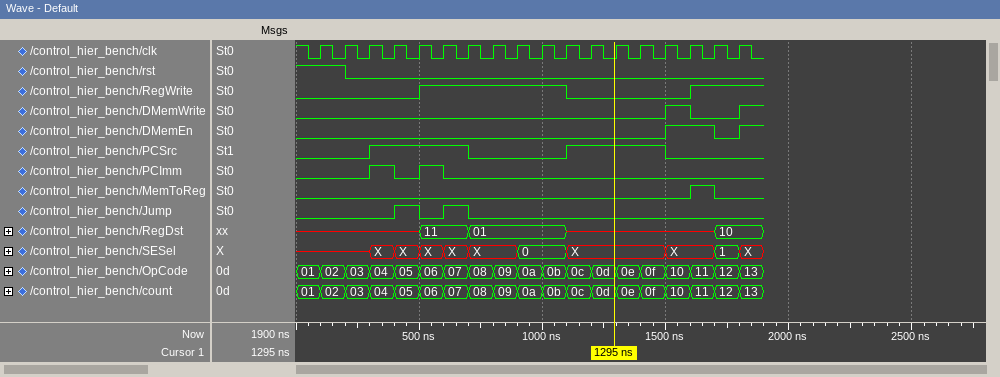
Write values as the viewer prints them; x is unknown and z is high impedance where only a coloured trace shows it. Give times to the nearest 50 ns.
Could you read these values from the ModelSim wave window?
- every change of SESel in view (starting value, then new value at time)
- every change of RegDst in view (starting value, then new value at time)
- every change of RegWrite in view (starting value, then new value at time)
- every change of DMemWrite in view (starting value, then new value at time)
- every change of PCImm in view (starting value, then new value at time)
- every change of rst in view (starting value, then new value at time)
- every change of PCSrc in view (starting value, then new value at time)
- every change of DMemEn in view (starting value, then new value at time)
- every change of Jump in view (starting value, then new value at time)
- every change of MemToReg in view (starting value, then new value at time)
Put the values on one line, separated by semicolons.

x, X at 300 ns, X at 400 ns, X at 500 ns, X at 600 ns, X at 700 ns, 0 at 900 ns, X at 1100 ns, X at 1500 ns, 1 at 1700 ns, X at 1800 ns; x, 11 at 500 ns, 01 at 700 ns, x at 1100 ns, 10 at 1700 ns; 0, 1 at 500 ns, 0 at 1100 ns, 1 at 1600 ns; 0, 1 at 1500 ns, 0 at 1600 ns, 1 at 1800 ns; 0, 1 at 300 ns, 0 at 400 ns, 1 at 500 ns, 0 at 600 ns; 1, 0 at 200 ns; 0, 1 at 300 ns, 0 at 700 ns, 1 at 1100 ns, 0 at 1500 ns; 0, 1 at 1500 ns, 0 at 1700 ns, 1 at 1800 ns; 0, 1 at 400 ns, 0 at 500 ns, 1 at 600 ns, 0 at 700 ns; 0, 1 at 1600 ns, 0 at 1700 ns
